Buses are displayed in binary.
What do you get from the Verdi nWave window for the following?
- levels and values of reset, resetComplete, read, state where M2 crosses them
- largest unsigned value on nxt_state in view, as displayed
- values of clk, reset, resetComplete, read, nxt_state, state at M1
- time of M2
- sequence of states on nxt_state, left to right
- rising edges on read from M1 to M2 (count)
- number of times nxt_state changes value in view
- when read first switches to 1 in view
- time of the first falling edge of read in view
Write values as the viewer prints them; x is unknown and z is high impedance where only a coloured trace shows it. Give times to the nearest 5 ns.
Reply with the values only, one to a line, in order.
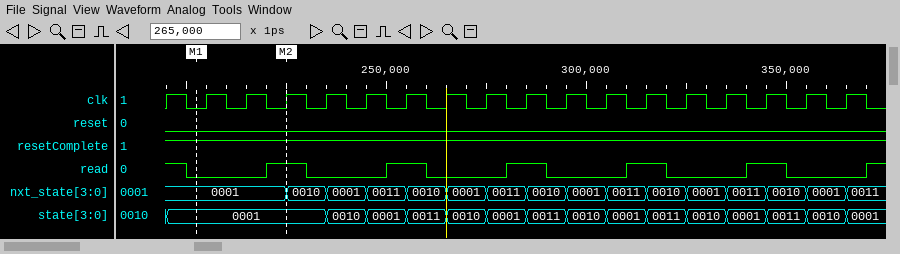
reset=0, resetComplete=1, read=1, state=0001
0011
clk=0, reset=0, resetComplete=1, read=0, nxt_state=0001, state=0001
225 ns
0001, 0010, 0001, 0011, 0010, 0001, 0011, 0010, 0001, 0011, 0010, 0001, 0011, 0010, 0001, 0011
1
15
220 ns
200 ns
